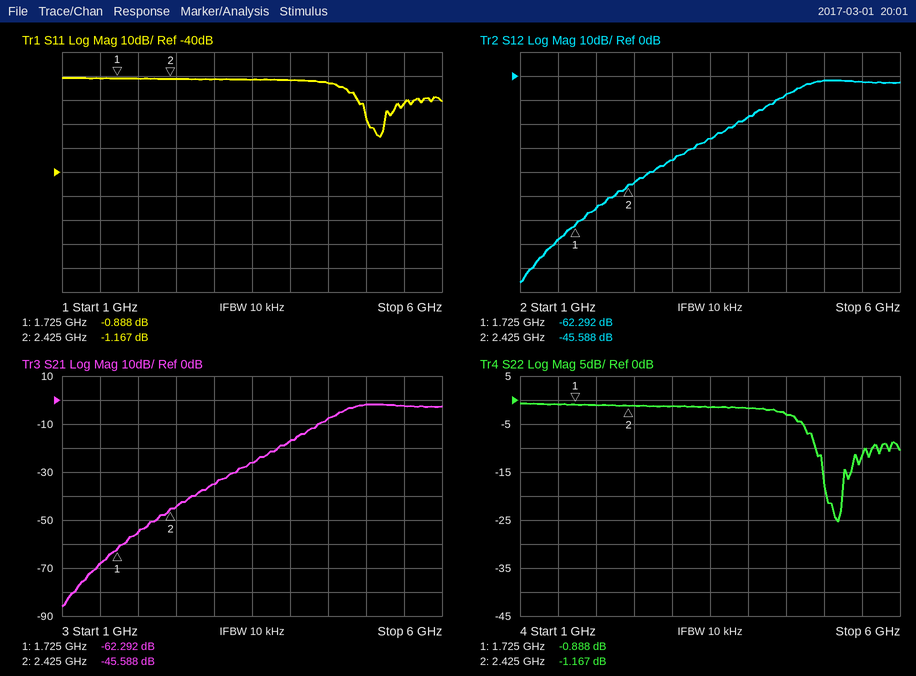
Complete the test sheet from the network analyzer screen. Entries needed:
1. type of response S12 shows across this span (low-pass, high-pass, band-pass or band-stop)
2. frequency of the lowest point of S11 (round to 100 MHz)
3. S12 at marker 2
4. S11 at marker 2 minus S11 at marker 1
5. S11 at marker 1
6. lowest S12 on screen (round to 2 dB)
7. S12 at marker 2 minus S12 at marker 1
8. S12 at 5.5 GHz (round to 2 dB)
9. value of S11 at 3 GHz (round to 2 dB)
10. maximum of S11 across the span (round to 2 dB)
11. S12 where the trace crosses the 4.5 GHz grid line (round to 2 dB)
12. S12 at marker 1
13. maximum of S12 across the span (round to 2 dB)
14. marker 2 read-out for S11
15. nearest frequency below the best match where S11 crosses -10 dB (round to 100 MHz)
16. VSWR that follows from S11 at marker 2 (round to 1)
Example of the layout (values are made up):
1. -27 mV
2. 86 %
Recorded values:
1. high-pass
2. 5.2 GHz
3. -45.588 dB
4. -0.279 dB
5. -0.888 dB
6. -86 dB
7. 16.704 dB
8. -2 dB
9. -2 dB
10. 0 dB
11. -8 dB
12. -62.292 dB
13. -2 dB
14. -1.167 dB
15. 4.9 GHz
16. 15
